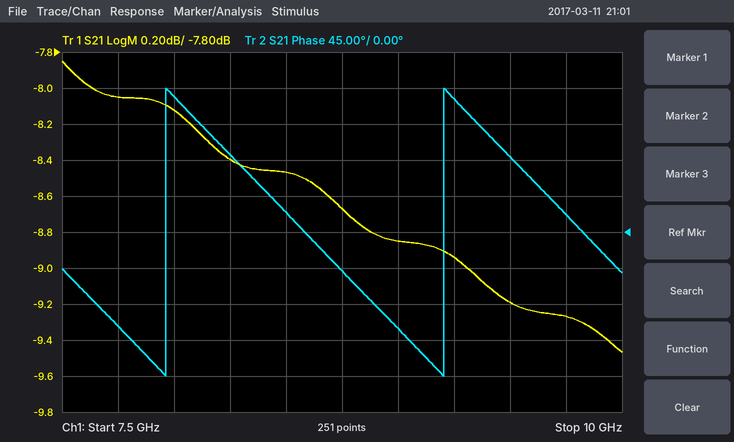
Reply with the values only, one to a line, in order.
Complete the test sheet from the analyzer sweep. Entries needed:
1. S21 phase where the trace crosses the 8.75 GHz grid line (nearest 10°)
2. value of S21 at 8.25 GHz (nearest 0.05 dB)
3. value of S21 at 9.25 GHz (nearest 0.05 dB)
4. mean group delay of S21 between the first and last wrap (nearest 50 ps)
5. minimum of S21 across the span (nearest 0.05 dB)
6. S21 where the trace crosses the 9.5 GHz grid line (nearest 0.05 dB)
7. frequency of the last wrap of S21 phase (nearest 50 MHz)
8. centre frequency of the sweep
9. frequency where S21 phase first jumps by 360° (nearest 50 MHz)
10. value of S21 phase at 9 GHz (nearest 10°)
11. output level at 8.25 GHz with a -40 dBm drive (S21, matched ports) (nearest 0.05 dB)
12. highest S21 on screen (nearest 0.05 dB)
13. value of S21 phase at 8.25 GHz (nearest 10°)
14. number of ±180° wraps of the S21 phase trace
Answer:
-50°
-8.40 dB
-8.95 dB
800 ps
-9.45 dB
-9.20 dB
9.20 GHz
8.75 GHz
7.95 GHz
-120°
-48.40 dBm
-7.85 dB
100°
2
